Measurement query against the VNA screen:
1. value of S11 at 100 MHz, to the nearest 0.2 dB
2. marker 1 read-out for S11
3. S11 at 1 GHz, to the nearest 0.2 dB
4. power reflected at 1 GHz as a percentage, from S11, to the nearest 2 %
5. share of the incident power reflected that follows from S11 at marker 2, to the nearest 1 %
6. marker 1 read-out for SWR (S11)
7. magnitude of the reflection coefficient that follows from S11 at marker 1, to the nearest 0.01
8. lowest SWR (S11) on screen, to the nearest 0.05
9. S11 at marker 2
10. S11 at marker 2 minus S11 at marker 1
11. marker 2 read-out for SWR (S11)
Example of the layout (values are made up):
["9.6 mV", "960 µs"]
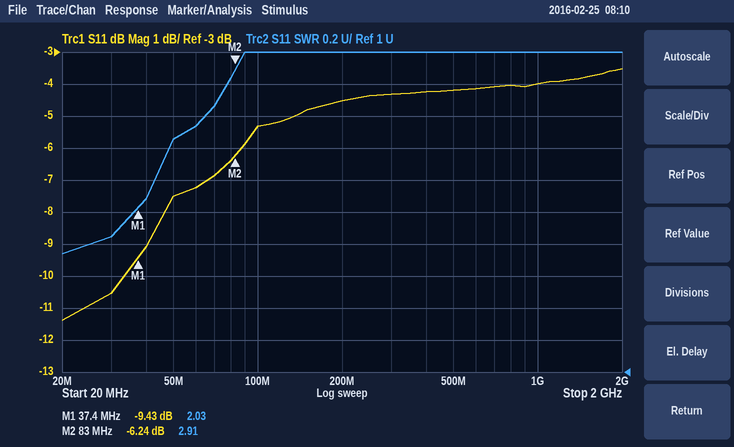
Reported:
["-5.4 dB", "-9.43 dB", "-4.0 dB", "40 %", "24 %", "2.03", "0.34", "1.75", "-6.24 dB", "3.19 dB", "2.91"]
